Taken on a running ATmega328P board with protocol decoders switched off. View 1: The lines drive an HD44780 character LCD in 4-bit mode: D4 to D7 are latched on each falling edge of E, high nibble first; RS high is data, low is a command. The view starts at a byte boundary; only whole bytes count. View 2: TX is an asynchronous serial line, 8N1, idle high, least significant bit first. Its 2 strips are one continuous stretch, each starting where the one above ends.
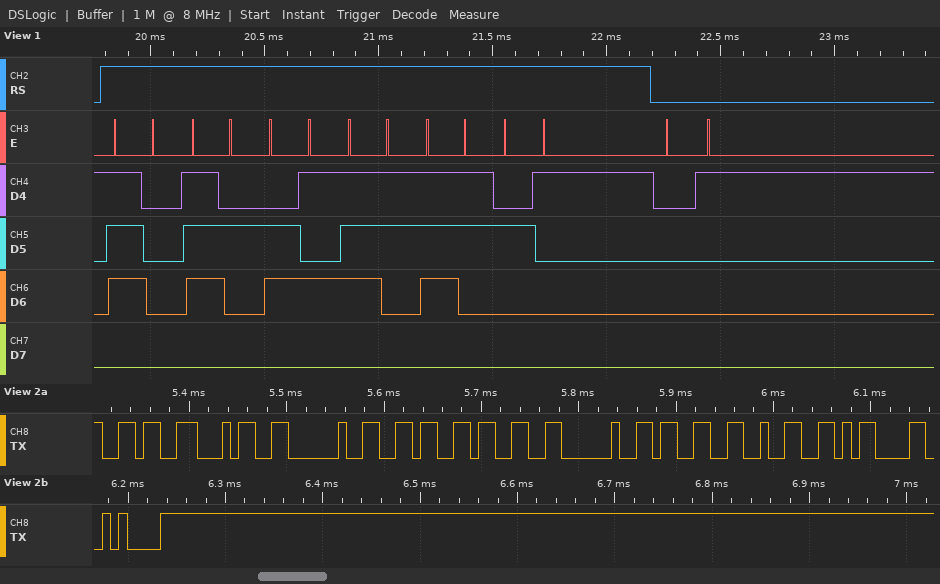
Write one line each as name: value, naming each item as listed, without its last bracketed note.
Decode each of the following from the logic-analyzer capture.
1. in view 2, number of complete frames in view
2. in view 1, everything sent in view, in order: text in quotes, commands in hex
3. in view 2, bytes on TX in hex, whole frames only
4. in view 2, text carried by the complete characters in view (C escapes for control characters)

in view 2, number of complete frames in view: 10
in view 1, everything sent in view, in order: text in quotes, commands in hex: "press!" 0x01
in view 2, bytes on TX in hex, whole frames only: 0x36 0x34 0x20 0x36 0x33 0x20 0x33 0x32 0x0D 0x0A
in view 2, text carried by the complete characters in view: "64 63 32\r\n"
